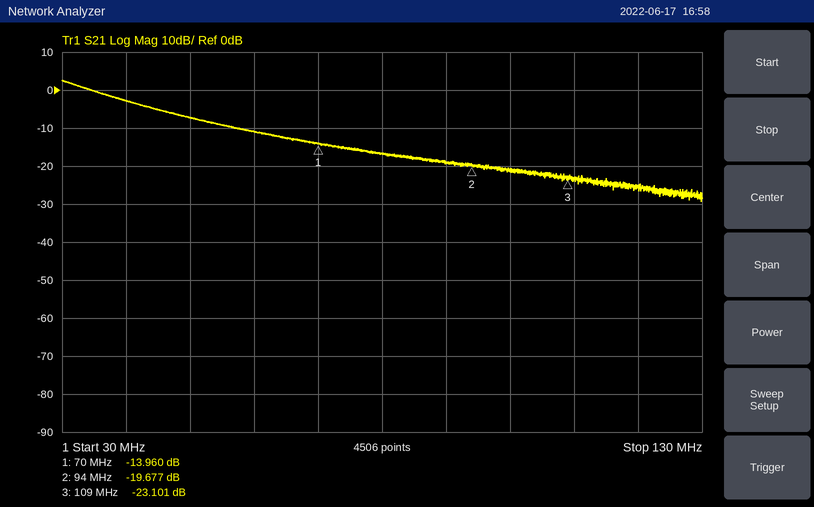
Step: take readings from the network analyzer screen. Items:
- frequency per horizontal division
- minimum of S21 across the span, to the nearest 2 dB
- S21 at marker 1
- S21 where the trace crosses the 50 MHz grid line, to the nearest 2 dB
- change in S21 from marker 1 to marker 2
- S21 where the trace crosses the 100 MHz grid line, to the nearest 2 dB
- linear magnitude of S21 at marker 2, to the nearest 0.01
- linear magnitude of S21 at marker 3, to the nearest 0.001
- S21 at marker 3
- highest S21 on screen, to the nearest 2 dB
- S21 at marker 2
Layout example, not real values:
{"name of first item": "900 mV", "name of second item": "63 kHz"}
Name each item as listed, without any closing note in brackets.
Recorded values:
{"frequency per horizontal division": "10 MHz", "minimum of S21 across the span, to the nearest 2 dB": "-30 dB", "S21 at marker 1": "-13.960 dB", "S21 where the trace crosses the 50 MHz grid line, to the nearest 2 dB": "-8 dB", "change in S21 from marker 1 to marker 2": "-5.717 dB", "S21 where the trace crosses the 100 MHz grid line, to the nearest 2 dB": "-22 dB", "linear magnitude of S21 at marker 2, to the nearest 0.01": "0.10", "linear magnitude of S21 at marker 3, to the nearest 0.001": "0.070", "S21 at marker 3": "-23.101 dB", "highest S21 on screen, to the nearest 2 dB": "2 dB", "S21 at marker 2": "-19.677 dB"}
